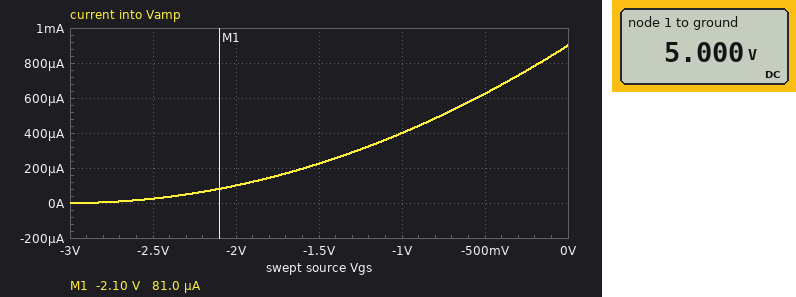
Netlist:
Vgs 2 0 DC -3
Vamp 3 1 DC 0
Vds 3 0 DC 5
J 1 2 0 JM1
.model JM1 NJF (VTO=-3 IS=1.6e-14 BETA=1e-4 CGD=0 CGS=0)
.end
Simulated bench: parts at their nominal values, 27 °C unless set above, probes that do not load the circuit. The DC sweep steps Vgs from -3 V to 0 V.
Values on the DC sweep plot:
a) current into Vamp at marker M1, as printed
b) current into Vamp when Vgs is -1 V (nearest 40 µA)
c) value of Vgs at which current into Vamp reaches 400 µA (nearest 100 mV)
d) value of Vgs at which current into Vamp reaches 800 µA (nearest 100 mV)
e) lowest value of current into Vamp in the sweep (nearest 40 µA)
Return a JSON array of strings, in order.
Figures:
["81.0 µA", "400 µA", "-1.0 V", "-200 mV", "0 A"]
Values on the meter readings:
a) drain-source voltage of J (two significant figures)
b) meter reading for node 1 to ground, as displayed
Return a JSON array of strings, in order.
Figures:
["5.0 V", "5.000 V"]
